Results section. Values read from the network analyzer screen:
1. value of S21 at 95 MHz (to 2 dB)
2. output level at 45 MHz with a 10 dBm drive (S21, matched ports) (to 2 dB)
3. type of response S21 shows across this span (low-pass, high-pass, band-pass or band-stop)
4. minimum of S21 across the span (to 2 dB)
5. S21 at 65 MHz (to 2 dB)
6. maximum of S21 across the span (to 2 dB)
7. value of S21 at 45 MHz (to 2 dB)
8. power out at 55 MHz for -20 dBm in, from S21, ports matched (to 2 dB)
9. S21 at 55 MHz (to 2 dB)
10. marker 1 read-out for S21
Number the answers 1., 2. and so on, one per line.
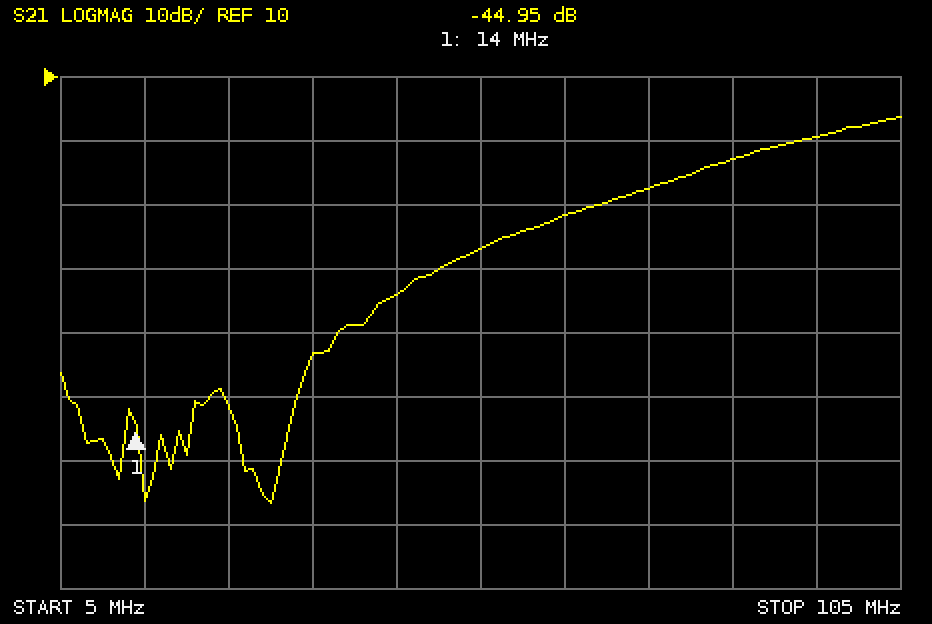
1. 0 dB
2. -14 dBm
3. high-pass
4. -56 dB
5. -12 dB
6. 4 dB
7. -24 dB
8. -36 dBm
9. -16 dB
10. -44.95 dB
